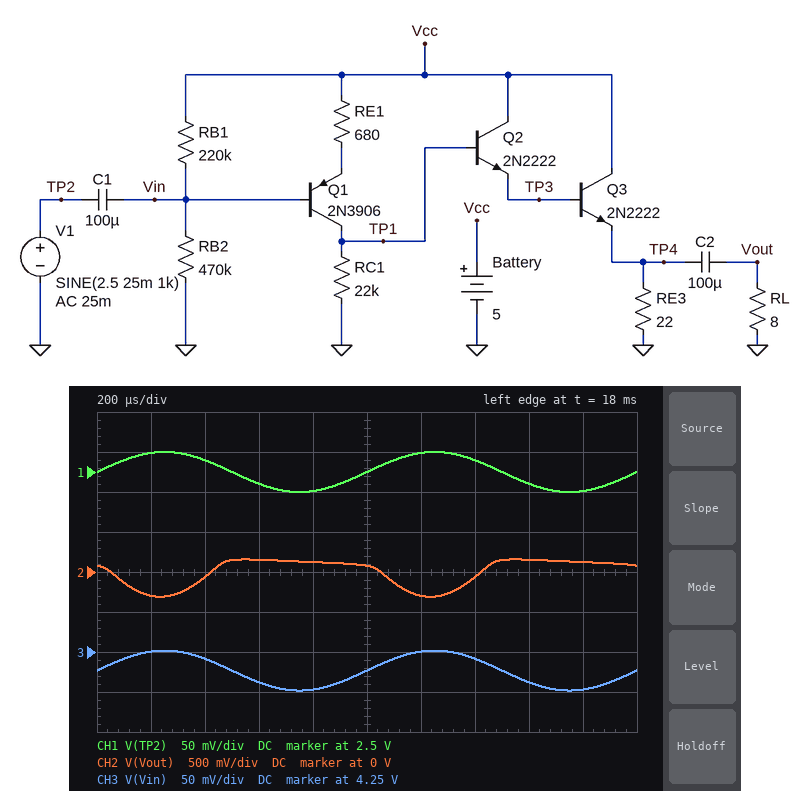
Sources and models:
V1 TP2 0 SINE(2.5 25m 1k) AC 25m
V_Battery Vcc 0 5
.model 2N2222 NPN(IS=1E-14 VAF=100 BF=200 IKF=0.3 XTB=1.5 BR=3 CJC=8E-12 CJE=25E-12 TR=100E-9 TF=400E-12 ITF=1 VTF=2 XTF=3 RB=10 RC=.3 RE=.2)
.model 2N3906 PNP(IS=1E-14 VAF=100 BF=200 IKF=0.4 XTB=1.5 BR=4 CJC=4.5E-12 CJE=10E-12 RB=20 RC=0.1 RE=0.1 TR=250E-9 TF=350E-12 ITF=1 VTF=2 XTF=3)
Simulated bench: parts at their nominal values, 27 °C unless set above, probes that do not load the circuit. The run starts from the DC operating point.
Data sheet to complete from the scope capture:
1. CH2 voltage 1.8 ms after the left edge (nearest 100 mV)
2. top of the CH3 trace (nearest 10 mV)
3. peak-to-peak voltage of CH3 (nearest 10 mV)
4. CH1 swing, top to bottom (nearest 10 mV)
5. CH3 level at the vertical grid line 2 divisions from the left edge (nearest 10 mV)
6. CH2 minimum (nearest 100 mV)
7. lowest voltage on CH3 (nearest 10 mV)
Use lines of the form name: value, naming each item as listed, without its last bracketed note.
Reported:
CH2 voltage 1.8 ms after the left edge: 100 mV
top of the CH3 trace: 4.25 V
peak-to-peak voltage of CH3: 50 mV
CH1 swing, top to bottom: 50 mV
CH3 level at the vertical grid line 2 divisions from the left edge: 4.24 V
CH2 minimum: -300 mV
lowest voltage on CH3: 4.20 V
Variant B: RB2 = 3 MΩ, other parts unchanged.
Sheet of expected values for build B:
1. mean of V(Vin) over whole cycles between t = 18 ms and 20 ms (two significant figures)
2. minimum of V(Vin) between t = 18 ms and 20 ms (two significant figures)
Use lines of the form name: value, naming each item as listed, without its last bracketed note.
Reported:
mean of V(Vin) over whole cycles between t = 18 ms and 20 ms: 4.7 V
minimum of V(Vin) between t = 18 ms and 20 ms: 4.6 V
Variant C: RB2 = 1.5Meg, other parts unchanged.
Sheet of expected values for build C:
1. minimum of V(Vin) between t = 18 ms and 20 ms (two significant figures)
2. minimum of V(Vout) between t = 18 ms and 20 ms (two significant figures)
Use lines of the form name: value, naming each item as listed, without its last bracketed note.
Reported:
minimum of V(Vin) between t = 18 ms and 20 ms: 4.4 V
minimum of V(Vout) between t = 18 ms and 20 ms: -11 mV
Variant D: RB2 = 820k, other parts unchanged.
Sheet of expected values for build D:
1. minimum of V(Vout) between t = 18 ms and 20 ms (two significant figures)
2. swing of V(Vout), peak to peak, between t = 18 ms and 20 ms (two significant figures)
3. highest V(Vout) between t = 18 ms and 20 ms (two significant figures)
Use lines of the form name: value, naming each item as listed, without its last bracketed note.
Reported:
minimum of V(Vout) between t = 18 ms and 20 ms: -380 mV
swing of V(Vout), peak to peak, between t = 18 ms and 20 ms: 610 mV
highest V(Vout) between t = 18 ms and 20 ms: 230 mV
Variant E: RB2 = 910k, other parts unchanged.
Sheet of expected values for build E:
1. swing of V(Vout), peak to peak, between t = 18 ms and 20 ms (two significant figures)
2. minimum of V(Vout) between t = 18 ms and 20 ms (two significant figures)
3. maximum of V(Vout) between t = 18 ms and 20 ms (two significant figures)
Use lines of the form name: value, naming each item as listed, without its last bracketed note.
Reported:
swing of V(Vout), peak to peak, between t = 18 ms and 20 ms: 660 mV
minimum of V(Vout) between t = 18 ms and 20 ms: -400 mV
maximum of V(Vout) between t = 18 ms and 20 ms: 260 mV
